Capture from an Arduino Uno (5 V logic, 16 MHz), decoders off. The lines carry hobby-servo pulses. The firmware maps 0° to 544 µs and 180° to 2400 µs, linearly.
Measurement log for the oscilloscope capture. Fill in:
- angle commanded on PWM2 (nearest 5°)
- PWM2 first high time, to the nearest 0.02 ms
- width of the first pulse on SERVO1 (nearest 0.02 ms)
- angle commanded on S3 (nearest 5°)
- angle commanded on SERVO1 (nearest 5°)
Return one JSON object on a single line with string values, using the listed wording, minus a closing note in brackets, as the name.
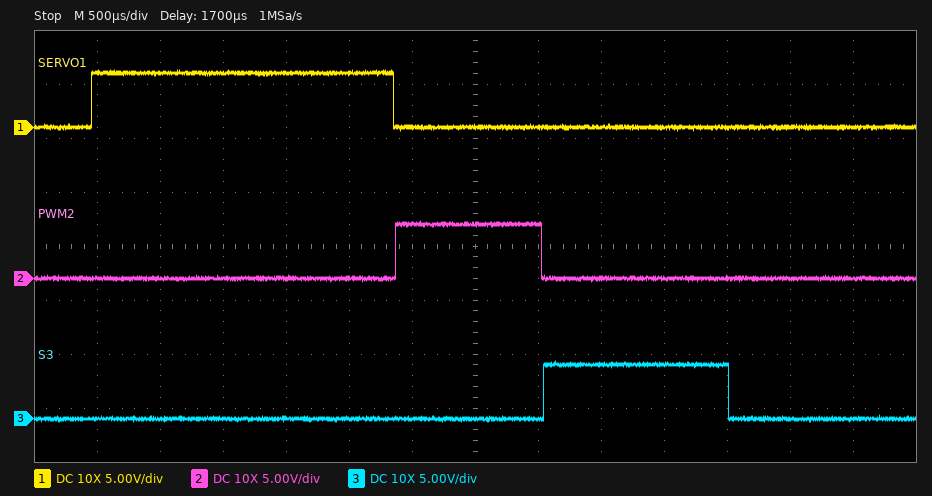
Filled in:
{"angle commanded on PWM2": "60°", "PWM2 first high time, to the nearest 0.02 ms": "1.16 ms", "width of the first pulse on SERVO1": "2.40 ms", "angle commanded on S3": "90°", "angle commanded on SERVO1": "180°"}
